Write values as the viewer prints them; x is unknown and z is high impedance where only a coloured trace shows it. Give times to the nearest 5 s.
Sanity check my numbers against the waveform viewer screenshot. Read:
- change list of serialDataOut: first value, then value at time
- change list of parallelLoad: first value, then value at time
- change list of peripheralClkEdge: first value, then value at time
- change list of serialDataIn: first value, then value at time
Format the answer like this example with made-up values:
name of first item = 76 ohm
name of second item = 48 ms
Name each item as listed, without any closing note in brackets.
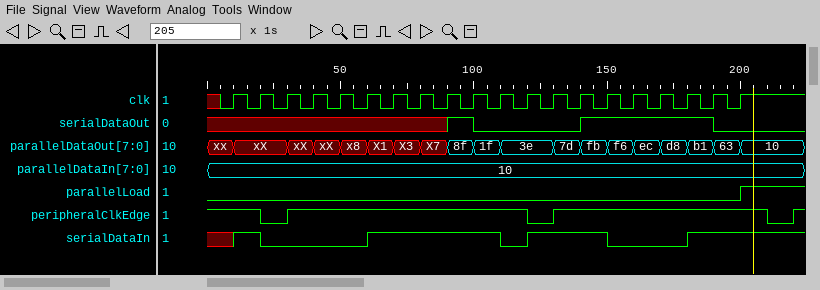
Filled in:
change list of serialDataOut: first value, then value at time = x, 1 at 90 s, 0 at 100 s, 1 at 140 s, 0 at 190 s
change list of parallelLoad: first value, then value at time = 0, 1 at 200 s
change list of peripheralClkEdge: first value, then value at time = 1, 0 at 20 s, 1 at 30 s, 0 at 120 s, 1 at 130 s, 0 at 210 s, 1 at 220 s
change list of serialDataIn: first value, then value at time = x, 1 at 10 s, 0 at 20 s, 1 at 60 s, 0 at 110 s, 1 at 120 s, 0 at 150 s, 1 at 180 s
